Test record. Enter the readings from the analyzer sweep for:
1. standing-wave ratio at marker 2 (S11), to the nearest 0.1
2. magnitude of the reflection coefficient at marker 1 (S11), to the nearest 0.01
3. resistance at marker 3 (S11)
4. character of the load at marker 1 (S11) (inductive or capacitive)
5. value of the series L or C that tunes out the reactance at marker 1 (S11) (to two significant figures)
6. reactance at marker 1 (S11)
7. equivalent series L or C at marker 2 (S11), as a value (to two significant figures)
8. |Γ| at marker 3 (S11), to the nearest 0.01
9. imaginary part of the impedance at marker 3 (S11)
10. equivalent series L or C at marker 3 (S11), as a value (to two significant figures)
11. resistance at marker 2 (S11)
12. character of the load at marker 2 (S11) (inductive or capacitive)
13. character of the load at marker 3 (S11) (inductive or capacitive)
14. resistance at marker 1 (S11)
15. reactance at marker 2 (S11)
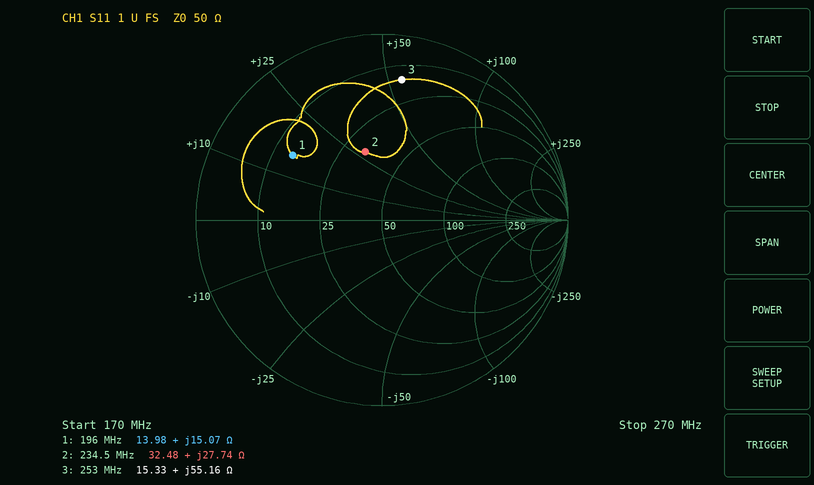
2.2
0.59
15.33 Ω
inductive
54 pF
+15.07 Ω
19 nH
0.76
+55.16 Ω
35 nH
32.48 Ω
inductive
inductive
13.98 Ω
+27.74 Ω
